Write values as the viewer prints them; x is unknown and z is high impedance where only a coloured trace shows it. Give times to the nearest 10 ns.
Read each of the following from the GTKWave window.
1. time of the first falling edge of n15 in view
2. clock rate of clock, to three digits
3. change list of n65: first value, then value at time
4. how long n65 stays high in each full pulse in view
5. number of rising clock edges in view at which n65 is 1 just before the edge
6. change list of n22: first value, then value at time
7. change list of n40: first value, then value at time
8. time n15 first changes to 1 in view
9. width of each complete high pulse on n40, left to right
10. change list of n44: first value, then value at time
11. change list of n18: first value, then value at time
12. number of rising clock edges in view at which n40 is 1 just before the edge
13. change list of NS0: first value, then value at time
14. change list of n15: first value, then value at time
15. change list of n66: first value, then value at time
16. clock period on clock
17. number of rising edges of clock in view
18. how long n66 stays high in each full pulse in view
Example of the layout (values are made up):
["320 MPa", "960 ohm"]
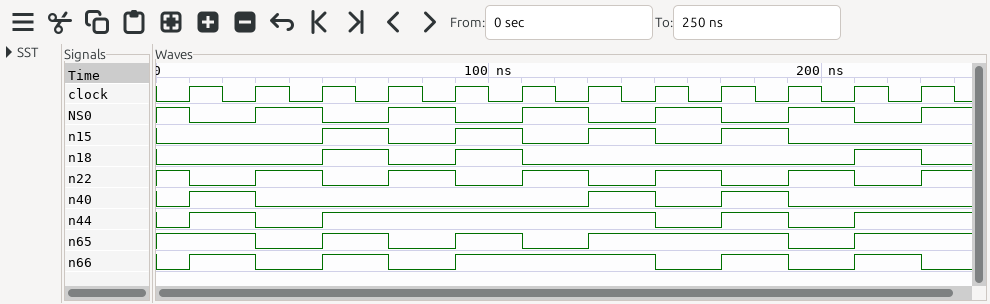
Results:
["70 ns", "50.0 MHz", "1, 0 at 30 ns, 1 at 50 ns, 0 at 70 ns, 1 at 90 ns, 0 at 110 ns, 1 at 130 ns, 0 at 190 ns, 1 at 210 ns", "20 ns, 20 ns, 60 ns", "8", "1, 0 at 10 ns, 1 at 30 ns, 0 at 50 ns, 1 at 70 ns, 0 at 90 ns, 1 at 110 ns, 0 at 130 ns, 1 at 150 ns, 0 at 170 ns, 1 at 190 ns, 0 at 210 ns, 1 at 230 ns", "0, 1 at 10 ns, 0 at 30 ns, 1 at 130 ns, 0 at 150 ns, 1 at 170 ns, 0 at 190 ns", "50 ns", "20 ns, 20 ns, 20 ns", "0, 1 at 10 ns, 0 at 30 ns, 1 at 50 ns, 0 at 150 ns, 1 at 170 ns, 0 at 190 ns, 1 at 210 ns", "0, 1 at 50 ns, 0 at 70 ns, 1 at 90 ns, 0 at 110 ns, 1 at 210 ns, 0 at 230 ns", "3", "1, 0 at 10 ns, 1 at 30 ns, 0 at 50 ns, 1 at 70 ns, 0 at 90 ns, 1 at 110 ns, 0 at 130 ns, 1 at 150 ns, 0 at 170 ns, 1 at 190 ns, 0 at 210 ns, 1 at 230 ns", "0, 1 at 50 ns, 0 at 70 ns, 1 at 90 ns, 0 at 110 ns, 1 at 130 ns, 0 at 150 ns, 1 at 170 ns, 0 at 190 ns", "0, 1 at 10 ns, 0 at 30 ns, 1 at 50 ns, 0 at 70 ns, 1 at 90 ns, 0 at 150 ns, 1 at 170 ns, 0 at 190 ns, 1 at 210 ns, 0 at 230 ns", "20 ns", "12", "20 ns, 20 ns, 60 ns, 20 ns, 20 ns"]
